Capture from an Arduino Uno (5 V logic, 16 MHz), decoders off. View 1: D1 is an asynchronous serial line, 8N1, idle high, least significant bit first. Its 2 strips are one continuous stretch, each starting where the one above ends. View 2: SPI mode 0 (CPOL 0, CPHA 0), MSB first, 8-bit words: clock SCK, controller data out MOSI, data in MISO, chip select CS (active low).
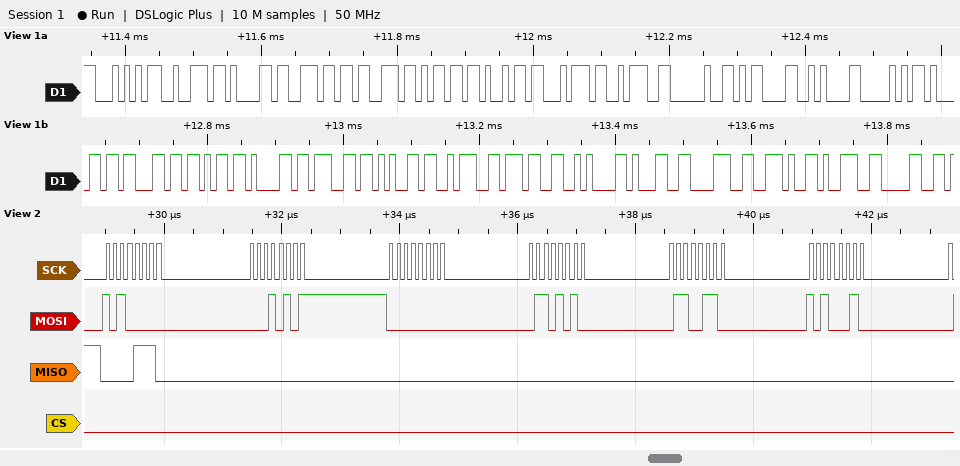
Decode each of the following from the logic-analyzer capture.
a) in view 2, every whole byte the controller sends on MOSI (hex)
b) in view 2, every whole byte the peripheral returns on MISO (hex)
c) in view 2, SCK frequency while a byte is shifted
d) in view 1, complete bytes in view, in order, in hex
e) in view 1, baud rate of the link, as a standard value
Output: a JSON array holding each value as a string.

["A0 15 00 6A 66 A2", "0E 00 00 00 00 00", "8 MHz", "54 72 61 6E 73 6D 69 74 3A 20 0D 0A 50 61 63 6B 61 67 65 3A 37 0A 31 38 2E 39 30", "115200 baud"]
